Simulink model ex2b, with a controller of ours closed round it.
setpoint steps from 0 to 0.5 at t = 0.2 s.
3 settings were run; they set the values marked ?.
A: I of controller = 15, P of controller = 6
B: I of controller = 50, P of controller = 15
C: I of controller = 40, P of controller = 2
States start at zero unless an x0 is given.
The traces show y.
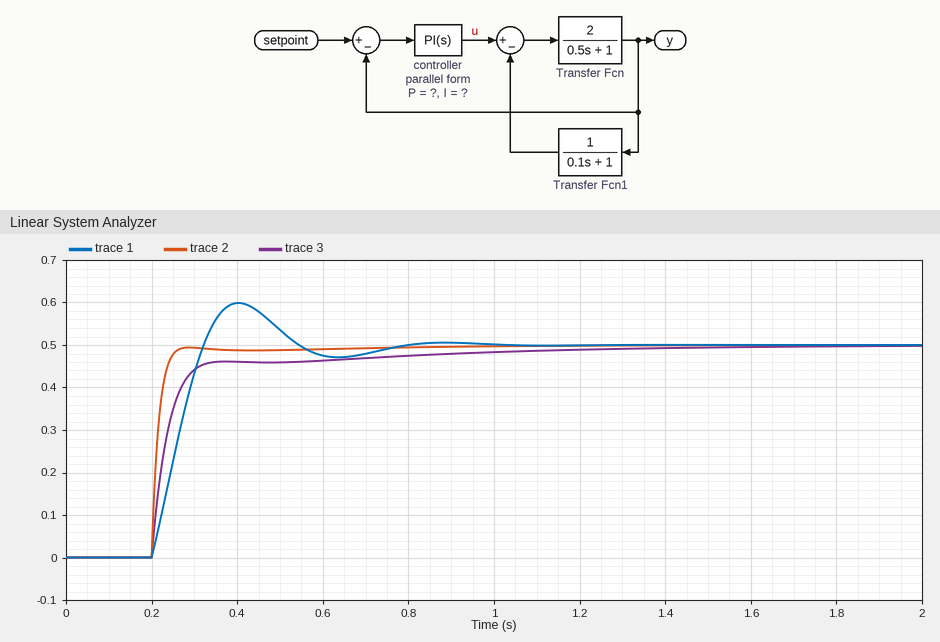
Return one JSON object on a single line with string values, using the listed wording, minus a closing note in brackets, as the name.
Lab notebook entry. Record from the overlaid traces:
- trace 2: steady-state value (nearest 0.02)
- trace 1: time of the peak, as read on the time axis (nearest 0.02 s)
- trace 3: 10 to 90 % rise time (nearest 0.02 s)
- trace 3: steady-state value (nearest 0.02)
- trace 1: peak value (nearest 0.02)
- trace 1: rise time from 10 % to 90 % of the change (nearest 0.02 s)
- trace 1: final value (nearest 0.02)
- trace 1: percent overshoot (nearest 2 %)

{"trace 2: steady-state value": "0.50", "trace 1: time of the peak, as read on the time axis": "0.40 s", "trace 3: 10 to 90 % rise time": "0.10 s", "trace 3: steady-state value": "0.50", "trace 1: peak value": "0.60", "trace 1: rise time from 10 % to 90 % of the change": "0.10 s", "trace 1: final value": "0.50", "trace 1: percent overshoot": "20 %"}
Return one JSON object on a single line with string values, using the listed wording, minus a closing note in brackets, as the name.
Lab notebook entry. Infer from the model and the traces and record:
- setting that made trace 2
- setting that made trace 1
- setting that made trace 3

{"setting that made trace 2": "B", "setting that made trace 1": "C", "setting that made trace 3": "A"}
